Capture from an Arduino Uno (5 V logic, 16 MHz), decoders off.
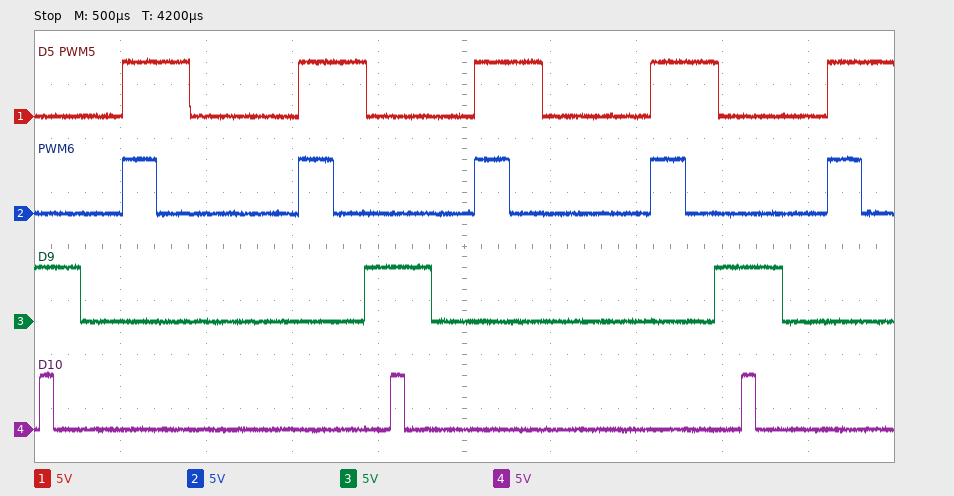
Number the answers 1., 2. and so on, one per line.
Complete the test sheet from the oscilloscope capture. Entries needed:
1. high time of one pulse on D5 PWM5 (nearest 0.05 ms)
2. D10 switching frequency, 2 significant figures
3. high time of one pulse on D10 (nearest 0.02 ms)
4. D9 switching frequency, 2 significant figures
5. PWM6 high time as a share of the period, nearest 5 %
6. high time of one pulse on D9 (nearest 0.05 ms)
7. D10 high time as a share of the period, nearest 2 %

1. 0.40 ms
2. 490 Hz
3. 0.08 ms
4. 490 Hz
5. 20 %
6. 0.40 ms
7. 4 %
